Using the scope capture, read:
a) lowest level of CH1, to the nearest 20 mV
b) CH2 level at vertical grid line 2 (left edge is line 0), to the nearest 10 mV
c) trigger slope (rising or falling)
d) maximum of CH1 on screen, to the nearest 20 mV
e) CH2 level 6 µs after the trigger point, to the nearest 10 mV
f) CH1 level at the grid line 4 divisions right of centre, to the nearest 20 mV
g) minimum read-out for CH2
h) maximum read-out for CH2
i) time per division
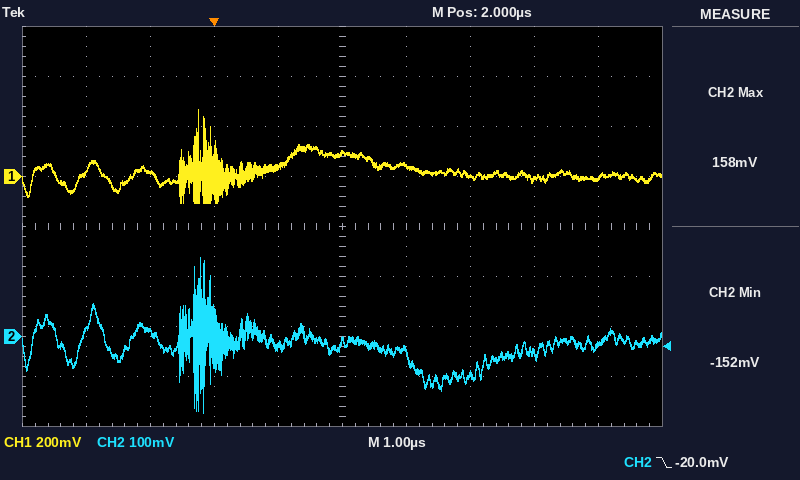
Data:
-100 mV
10 mV
falling
260 mV
-20 mV
0 mV
-152 mV
158 mV
1 µs
